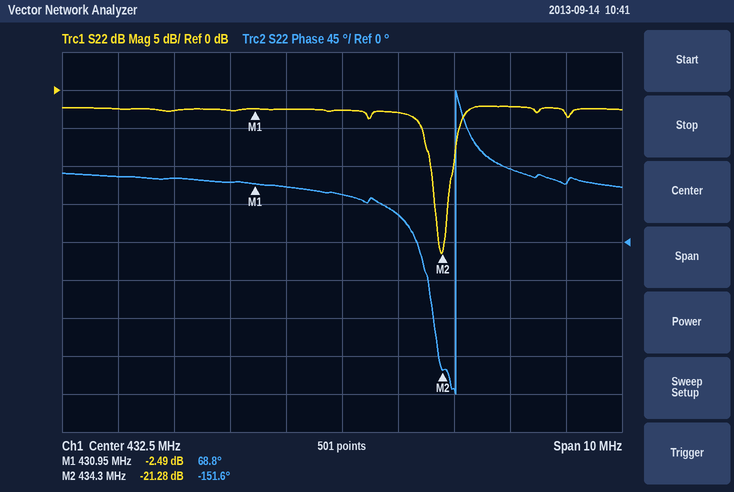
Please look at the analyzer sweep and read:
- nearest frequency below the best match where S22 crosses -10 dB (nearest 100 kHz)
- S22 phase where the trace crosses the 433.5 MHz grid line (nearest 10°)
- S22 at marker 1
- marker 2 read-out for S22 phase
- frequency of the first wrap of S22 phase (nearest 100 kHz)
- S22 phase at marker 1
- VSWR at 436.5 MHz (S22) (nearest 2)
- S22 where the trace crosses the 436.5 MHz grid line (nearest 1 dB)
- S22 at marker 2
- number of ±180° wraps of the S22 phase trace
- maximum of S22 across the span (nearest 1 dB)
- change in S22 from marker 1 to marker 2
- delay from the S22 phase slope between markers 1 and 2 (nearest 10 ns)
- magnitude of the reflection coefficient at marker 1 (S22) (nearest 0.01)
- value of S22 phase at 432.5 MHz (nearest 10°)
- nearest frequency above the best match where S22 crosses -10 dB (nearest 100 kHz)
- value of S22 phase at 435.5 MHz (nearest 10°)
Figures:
434.1 MHz
30°
-2.49 dB
-151.6°
434.5 MHz
68.8°
6
-3 dB
-21.28 dB
1
-2 dB
-18.79 dB
180 ns
0.75
60°
434.5 MHz
90°
